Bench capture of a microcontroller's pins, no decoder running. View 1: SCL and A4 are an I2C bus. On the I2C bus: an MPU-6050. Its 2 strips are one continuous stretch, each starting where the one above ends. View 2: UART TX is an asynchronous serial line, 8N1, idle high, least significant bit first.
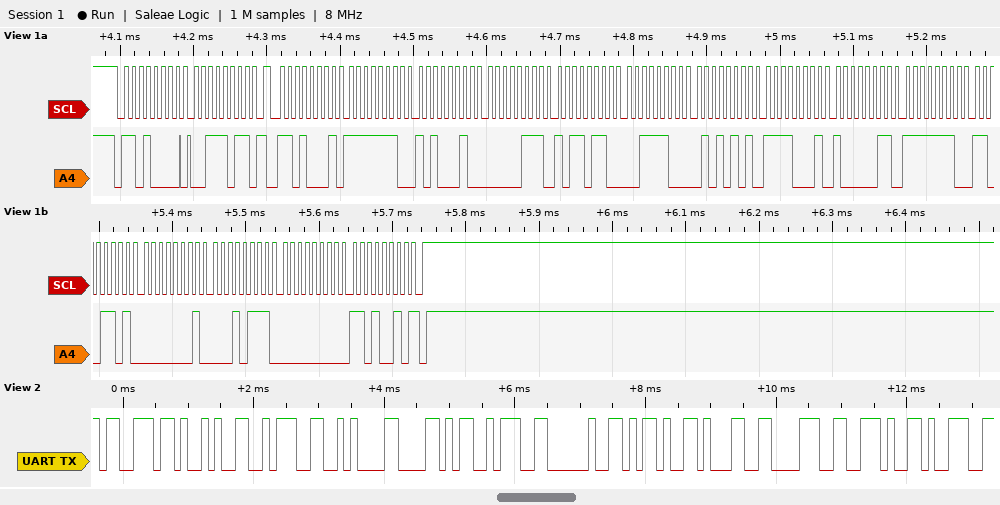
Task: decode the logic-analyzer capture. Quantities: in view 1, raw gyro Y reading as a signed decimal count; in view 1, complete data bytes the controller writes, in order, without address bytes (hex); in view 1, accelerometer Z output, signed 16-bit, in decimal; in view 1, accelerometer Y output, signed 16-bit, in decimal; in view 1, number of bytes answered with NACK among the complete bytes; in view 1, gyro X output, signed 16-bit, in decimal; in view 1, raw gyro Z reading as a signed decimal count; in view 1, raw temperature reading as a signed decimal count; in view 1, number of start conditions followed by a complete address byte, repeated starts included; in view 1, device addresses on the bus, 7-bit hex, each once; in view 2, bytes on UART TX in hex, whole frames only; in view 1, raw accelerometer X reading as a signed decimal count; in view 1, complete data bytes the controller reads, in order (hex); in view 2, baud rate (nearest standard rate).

279
3B
15445
1974
1
-307
210
-3709
2
0x68
0x73 0x29 0x3A 0x0A 0x58 0x3A 0x20 0x2D 0x31 0x38 0x2E 0x39
-350
FE A2 07 B6 3C 55 F1 83 FE CD 01 17 00 D2
9600 baud
